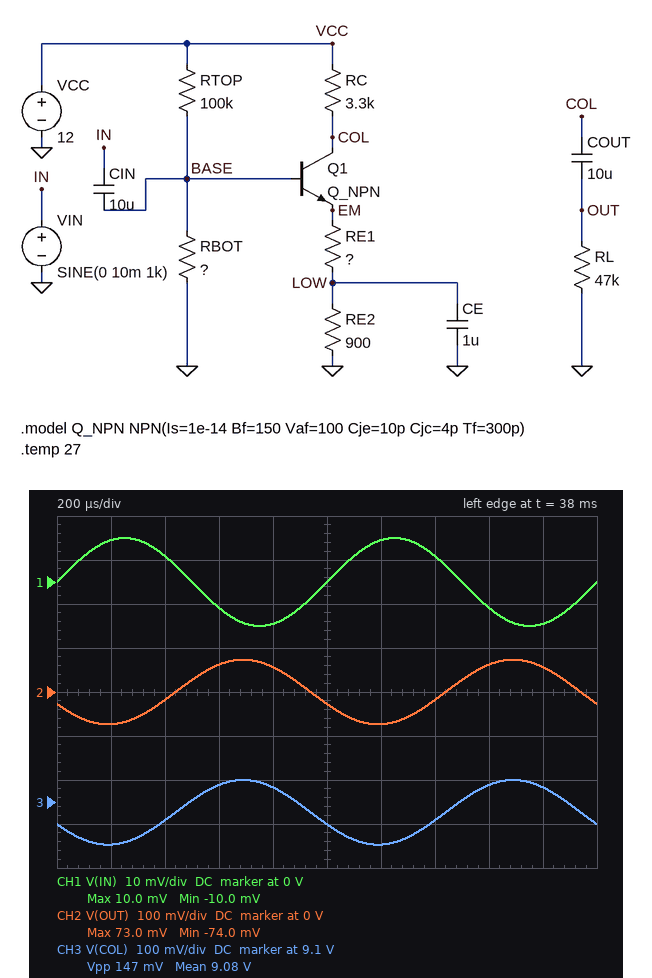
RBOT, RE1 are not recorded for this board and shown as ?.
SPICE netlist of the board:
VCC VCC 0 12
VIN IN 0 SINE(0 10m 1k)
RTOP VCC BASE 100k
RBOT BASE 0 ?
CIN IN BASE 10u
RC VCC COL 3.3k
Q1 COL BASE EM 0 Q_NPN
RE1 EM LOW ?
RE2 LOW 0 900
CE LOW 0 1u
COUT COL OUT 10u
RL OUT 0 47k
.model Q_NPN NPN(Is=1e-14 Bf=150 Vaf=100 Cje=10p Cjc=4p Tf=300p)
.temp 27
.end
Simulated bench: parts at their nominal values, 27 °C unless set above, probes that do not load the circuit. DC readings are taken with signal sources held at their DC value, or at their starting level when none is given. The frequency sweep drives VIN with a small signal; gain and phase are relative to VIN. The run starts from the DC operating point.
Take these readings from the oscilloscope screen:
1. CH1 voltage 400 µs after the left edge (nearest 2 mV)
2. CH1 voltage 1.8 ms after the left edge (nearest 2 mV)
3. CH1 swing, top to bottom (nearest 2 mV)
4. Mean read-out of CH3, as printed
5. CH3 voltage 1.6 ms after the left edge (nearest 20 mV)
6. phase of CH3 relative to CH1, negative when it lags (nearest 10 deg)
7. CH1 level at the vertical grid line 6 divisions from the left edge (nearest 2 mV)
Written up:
6 mV
-10 mV
20 mV
9.08 V
9.14 V
-160 deg
10 mV
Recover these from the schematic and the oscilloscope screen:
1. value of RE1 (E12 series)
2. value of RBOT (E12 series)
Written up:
330 Ω
18 kΩ
